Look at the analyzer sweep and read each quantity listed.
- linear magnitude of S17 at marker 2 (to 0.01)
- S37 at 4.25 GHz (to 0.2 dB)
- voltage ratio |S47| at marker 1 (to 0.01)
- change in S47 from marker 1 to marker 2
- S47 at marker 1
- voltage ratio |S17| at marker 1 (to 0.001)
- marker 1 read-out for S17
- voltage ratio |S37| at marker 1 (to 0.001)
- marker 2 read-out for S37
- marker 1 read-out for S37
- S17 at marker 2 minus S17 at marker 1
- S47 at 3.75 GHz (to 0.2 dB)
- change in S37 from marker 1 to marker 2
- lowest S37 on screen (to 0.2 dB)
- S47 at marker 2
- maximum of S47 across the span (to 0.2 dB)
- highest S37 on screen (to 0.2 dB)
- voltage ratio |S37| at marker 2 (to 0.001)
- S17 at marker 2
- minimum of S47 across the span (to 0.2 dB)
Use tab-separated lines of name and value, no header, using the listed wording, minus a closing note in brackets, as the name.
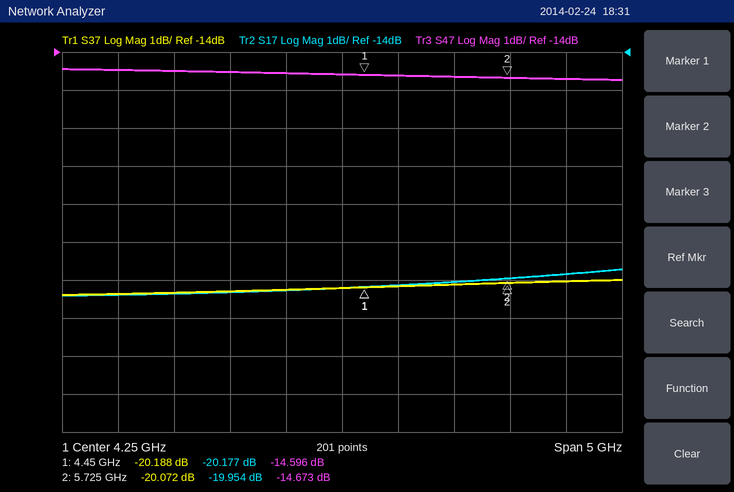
linear magnitude of S17 at marker 2	0.10
S37 at 4.25 GHz	-20.2 dB
voltage ratio |S47| at marker 1	0.19
change in S47 from marker 1 to marker 2	-0.077 dB
S47 at marker 1	-14.596 dB
voltage ratio |S17| at marker 1	0.098
marker 1 read-out for S17	-20.177 dB
voltage ratio |S37| at marker 1	0.098
marker 2 read-out for S37	-20.072 dB
marker 1 read-out for S37	-20.188 dB
S17 at marker 2 minus S17 at marker 1	0.223 dB
S47 at 3.75 GHz	-14.6 dB
change in S37 from marker 1 to marker 2	0.116 dB
lowest S37 on screen	-20.4 dB
S47 at marker 2	-14.673 dB
maximum of S47 across the span	-14.4 dB
highest S37 on screen	-20.0 dB
voltage ratio |S37| at marker 2	0.099
S17 at marker 2	-19.954 dB
minimum of S47 across the span	-14.8 dB
